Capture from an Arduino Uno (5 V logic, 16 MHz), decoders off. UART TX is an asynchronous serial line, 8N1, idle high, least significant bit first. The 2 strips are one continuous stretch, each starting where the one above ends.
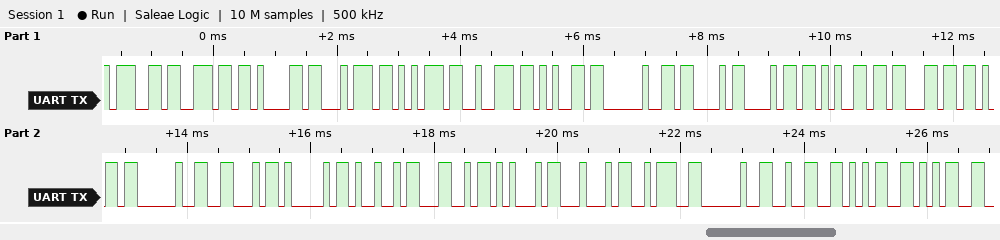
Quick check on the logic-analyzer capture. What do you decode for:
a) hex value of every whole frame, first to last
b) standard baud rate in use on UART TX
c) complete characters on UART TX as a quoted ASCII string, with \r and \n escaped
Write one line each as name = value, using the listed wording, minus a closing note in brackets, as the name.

hex value of every whole frame, first to last = 67 6E 61 74 75 72 65 20 43 68 65 63 6B 20 46 41 49 4C 45 44 3A 20 32 35 35
standard baud rate in use on UART TX = 9600 baud
complete characters on UART TX as a quoted ASCII string, with \r and \n escaped = "gnature Check FAILED: 255"
